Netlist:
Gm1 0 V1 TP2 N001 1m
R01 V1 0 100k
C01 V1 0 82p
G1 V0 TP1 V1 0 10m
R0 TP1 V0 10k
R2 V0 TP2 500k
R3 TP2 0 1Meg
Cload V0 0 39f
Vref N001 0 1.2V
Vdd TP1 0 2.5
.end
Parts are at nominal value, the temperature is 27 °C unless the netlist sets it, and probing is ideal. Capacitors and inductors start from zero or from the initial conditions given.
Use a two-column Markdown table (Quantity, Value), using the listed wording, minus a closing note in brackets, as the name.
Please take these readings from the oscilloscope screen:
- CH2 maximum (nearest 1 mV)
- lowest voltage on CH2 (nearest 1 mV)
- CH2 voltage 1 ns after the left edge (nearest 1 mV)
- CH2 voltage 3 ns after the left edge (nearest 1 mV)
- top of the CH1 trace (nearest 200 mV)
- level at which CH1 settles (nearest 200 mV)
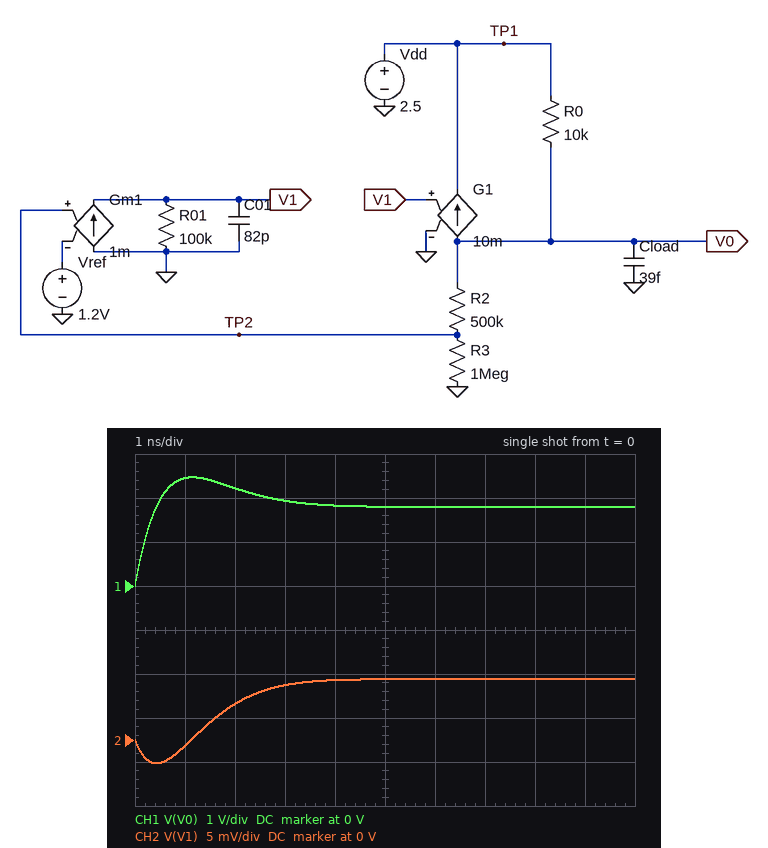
| Quantity | Value |
|---|---|
| CH2 maximum | 7 mV |
| lowest voltage on CH2 | -3 mV |
| CH2 voltage 1 ns after the left edge | -1 mV |
| CH2 voltage 3 ns after the left edge | 6 mV |
| top of the CH1 trace | 2.4 V |
| level at which CH1 settles | 1.8 V |
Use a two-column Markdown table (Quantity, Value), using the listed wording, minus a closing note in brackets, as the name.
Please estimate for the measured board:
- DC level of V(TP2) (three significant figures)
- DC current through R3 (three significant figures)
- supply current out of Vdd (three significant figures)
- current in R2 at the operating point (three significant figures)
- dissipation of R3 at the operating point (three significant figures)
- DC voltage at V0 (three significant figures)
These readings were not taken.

| Quantity | Value |
|---|---|
| DC level of V(TP2) | 1.20 V |
| DC current through R3 | 1.20 µA |
| supply current out of Vdd | 1.20 µA |
| current in R2 at the operating point | 1.20 µA |
| dissipation of R3 at the operating point | 1.44 µW |
| DC voltage at V0 | 1.80 V |
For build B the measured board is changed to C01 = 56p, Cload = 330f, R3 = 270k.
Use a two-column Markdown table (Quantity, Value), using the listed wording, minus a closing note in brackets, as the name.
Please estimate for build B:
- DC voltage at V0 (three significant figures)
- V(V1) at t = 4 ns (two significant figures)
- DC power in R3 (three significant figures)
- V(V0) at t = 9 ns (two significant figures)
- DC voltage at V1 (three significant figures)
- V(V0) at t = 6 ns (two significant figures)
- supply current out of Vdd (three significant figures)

| Quantity | Value |
|---|---|
| DC voltage at V0 | 3.42 V |
| V(V1) at t = 4 ns | -36 mV |
| DC power in R3 | 5.33 µW |
| V(V0) at t = 9 ns | 4.1 V |
| DC voltage at V1 | -9.66 mV |
| V(V0) at t = 6 ns | 4.6 V |
| supply current out of Vdd | 4.44 µA |
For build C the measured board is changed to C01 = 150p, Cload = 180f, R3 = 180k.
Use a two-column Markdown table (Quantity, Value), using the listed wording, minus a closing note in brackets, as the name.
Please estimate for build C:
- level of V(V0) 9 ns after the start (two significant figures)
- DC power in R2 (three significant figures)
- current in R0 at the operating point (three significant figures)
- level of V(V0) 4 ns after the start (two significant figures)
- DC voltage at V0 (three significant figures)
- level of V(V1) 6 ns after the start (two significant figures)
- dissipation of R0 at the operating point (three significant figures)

| Quantity | Value |
|---|---|
| level of V(V0) 9 ns after the start | 4.5 V |
| DC power in R2 | 22.2 µW |
| current in R0 at the operating point | 203 µA |
| level of V(V0) 4 ns after the start | 3.4 V |
| DC voltage at V0 | 4.53 V |
| level of V(V1) 6 ns after the start | -20 mV |
| dissipation of R0 at the operating point | 413 µW |
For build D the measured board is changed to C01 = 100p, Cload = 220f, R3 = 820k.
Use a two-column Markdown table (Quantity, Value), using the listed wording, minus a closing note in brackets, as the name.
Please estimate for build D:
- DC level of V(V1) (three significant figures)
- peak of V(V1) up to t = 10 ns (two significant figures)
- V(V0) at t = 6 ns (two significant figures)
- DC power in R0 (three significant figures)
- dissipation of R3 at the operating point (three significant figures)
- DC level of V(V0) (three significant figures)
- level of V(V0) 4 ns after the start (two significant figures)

| Quantity | Value |
|---|---|
| DC level of V(V1) | 5.54 mV |
| peak of V(V1) up to t = 10 ns | 9.2 mV |
| V(V0) at t = 6 ns | 2.5 V |
| DC power in R0 | 32.3 µW |
| dissipation of R3 at the operating point | 1.76 µW |
| DC level of V(V0) | 1.93 V |
| level of V(V0) 4 ns after the start | 2.7 V |
